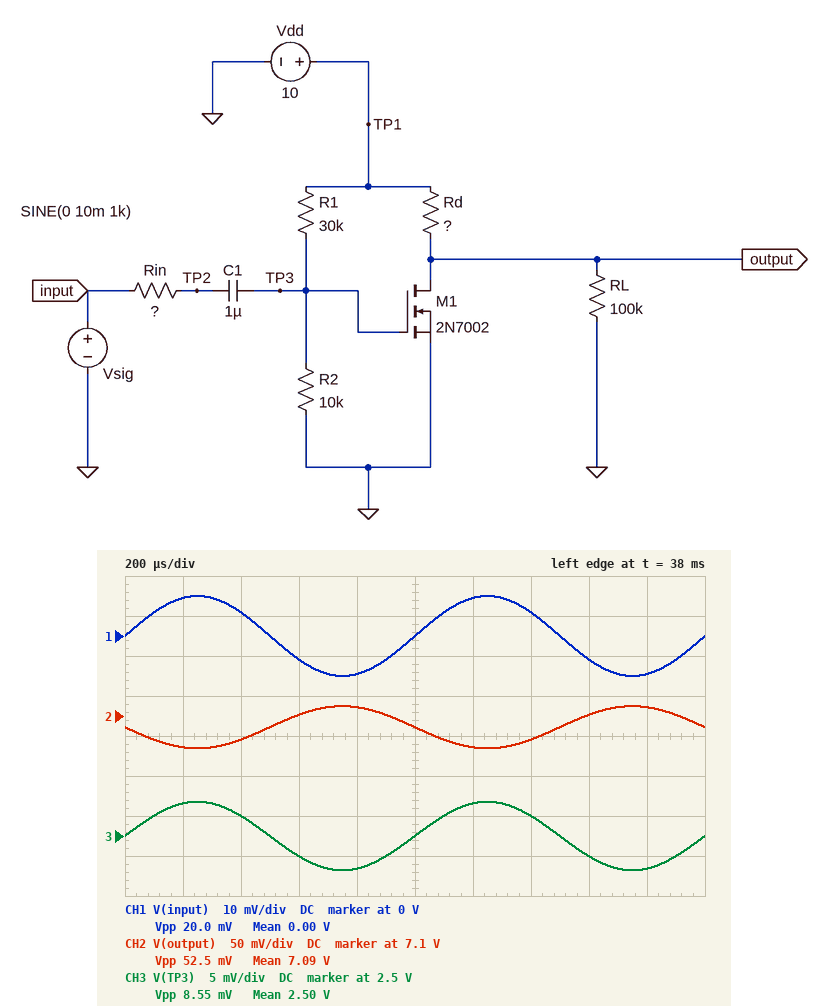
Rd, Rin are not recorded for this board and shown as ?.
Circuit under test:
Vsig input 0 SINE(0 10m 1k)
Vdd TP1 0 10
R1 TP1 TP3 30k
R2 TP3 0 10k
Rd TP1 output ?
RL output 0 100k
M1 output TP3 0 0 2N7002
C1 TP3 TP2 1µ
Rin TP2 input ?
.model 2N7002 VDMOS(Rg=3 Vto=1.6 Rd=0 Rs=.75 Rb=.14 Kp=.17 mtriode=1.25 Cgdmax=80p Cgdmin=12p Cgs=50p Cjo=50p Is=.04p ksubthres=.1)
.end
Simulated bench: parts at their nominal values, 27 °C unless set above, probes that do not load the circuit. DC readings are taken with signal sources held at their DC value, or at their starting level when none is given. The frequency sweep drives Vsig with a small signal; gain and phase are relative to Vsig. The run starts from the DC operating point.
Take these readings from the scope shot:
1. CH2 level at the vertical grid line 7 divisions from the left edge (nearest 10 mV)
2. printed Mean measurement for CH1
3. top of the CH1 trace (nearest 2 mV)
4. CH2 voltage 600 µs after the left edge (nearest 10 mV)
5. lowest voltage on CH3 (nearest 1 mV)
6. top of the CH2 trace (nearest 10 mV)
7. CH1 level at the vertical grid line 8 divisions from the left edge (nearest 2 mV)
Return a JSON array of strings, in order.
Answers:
["7.07 V", "0.00 V", "10 mV", "7.10 V", "2.496 V", "7.11 V", "-6 mV"]
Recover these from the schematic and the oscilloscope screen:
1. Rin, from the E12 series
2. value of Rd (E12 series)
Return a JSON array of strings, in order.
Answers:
["10 kΩ", "47 Ω"]
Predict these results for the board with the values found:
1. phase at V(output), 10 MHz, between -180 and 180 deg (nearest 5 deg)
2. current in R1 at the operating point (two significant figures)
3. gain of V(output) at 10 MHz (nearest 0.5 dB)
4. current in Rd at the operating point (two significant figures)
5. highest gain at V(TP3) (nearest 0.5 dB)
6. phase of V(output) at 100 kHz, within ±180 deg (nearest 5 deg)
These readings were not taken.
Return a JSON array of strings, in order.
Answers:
["90 deg", "250 µA", "-25.0 dB", "62 mA", "-7.5 dB", "155 deg"]
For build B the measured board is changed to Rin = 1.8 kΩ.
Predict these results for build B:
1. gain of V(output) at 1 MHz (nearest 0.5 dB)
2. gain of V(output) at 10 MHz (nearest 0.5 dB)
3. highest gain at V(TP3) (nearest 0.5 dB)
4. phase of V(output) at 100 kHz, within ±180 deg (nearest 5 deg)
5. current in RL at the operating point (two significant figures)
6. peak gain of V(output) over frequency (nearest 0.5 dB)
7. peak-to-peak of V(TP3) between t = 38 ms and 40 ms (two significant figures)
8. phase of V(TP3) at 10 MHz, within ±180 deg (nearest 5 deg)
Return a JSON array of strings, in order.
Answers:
["8.5 dB", "-10.0 dB", "-2.0 dB", "170 deg", "71 µA", "14.0 dB", "16 mV", "-80 deg"]
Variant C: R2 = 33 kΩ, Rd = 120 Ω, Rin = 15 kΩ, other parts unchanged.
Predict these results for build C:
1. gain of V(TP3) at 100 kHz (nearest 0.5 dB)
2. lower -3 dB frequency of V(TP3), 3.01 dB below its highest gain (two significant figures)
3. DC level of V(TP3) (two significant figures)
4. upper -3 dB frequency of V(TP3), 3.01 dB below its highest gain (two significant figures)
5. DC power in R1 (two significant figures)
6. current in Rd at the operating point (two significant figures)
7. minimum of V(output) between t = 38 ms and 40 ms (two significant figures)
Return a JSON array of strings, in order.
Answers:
["-7.5 dB", "5.2 Hz", "5.2 V", "160 kHz", "760 µW", "82 mA", "170 mV"]
